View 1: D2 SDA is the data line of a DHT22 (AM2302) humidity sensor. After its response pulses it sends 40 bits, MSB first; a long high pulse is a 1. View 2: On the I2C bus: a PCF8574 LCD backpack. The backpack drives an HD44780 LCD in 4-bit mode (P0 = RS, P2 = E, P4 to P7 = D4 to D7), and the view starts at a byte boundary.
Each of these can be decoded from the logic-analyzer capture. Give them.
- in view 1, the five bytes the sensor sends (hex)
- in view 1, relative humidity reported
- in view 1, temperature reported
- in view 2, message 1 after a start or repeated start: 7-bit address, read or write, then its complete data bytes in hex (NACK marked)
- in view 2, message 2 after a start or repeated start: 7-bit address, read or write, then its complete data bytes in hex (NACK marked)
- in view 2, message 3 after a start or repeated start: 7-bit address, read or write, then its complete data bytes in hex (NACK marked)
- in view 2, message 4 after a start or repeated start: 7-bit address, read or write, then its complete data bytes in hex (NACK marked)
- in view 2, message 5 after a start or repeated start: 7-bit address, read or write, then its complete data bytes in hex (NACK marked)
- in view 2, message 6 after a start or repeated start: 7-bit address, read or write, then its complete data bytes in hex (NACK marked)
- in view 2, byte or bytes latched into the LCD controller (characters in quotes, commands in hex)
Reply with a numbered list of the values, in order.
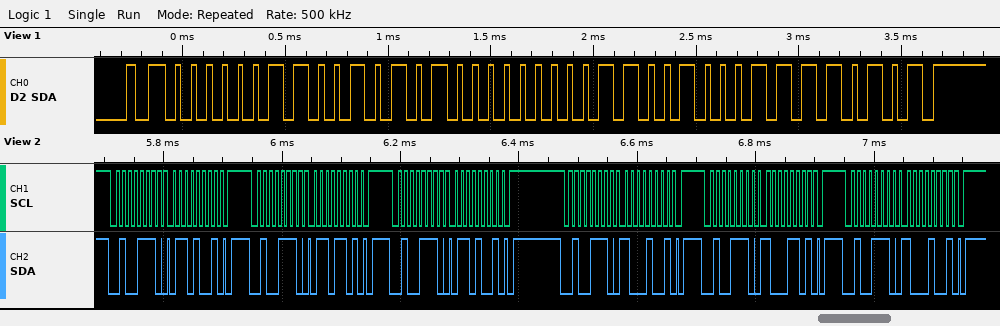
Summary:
1. 03 2A 00 C8 F5
2. 81.0 %
3. 20.0 °C
4. 0x27 write: 69
5. 0x27 write: 6D
6. 0x27 write: 69
7. 0x27 write: 89
8. 0x27 write: 8D
9. 0x27 write: 89
10. 'h'
